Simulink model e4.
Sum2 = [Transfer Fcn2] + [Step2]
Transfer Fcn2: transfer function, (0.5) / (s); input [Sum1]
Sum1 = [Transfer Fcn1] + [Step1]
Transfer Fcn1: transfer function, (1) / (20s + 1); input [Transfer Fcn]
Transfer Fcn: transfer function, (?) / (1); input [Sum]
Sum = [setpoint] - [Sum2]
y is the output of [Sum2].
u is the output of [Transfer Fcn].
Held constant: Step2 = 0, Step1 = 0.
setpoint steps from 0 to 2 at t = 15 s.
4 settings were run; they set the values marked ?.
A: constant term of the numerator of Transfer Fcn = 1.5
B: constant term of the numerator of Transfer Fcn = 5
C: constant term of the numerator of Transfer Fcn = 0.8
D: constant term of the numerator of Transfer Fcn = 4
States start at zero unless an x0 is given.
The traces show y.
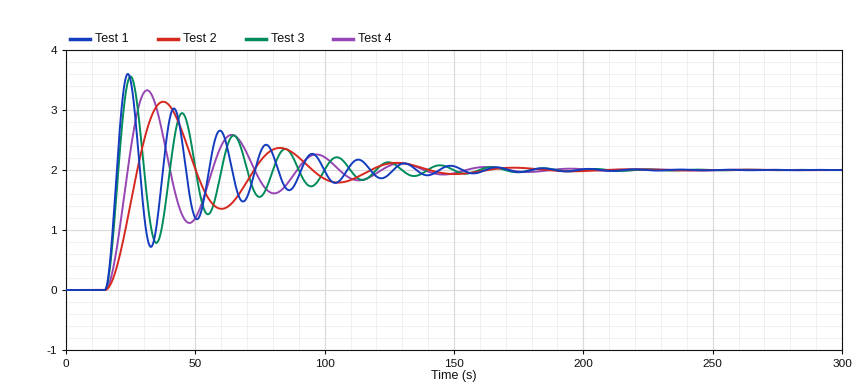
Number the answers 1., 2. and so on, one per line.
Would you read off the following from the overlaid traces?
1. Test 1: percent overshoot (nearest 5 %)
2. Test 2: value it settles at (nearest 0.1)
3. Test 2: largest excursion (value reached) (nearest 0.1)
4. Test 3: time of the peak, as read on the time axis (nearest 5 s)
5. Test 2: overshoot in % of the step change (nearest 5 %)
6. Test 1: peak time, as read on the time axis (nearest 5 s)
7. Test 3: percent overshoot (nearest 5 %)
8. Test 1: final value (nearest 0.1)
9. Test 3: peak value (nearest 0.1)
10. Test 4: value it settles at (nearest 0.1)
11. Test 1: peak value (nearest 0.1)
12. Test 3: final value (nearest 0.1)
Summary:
1. 80 %
2. 2.0
3. 3.1
4. 25 s
5. 55 %
6. 25 s
7. 80 %
8. 2.0
9. 3.6
10. 2.0
11. 3.6
12. 2.0
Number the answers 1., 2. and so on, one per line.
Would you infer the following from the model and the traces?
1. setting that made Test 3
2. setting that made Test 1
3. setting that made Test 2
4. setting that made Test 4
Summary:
1. D
2. B
3. C
4. A
